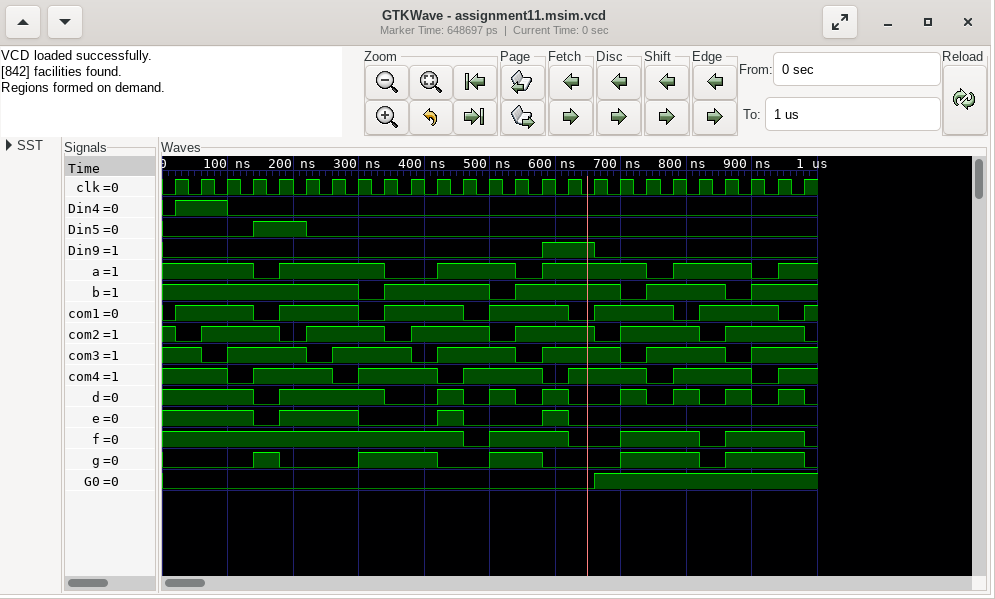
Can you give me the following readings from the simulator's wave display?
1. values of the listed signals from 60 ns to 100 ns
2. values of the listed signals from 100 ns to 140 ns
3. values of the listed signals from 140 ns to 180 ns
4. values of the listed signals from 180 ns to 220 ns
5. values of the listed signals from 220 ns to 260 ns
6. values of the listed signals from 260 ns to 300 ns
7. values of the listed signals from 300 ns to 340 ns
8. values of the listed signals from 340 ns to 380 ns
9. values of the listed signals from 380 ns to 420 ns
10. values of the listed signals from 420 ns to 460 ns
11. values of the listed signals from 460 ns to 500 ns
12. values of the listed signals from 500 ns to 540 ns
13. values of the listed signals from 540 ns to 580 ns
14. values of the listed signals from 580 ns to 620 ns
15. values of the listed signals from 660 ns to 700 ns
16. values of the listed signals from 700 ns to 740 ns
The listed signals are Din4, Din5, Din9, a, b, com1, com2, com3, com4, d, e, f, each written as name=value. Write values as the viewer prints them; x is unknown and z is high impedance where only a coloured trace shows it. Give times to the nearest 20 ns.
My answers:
Din4=1, Din5=0, Din9=0, a=1, b=1, com1=1, com2=1, com3=0, com4=1, d=1, e=1, f=1
Din4=0, Din5=0, Din9=0, a=1, b=1, com1=1, com2=1, com3=1, com4=0, d=1, e=1, f=1
Din4=0, Din5=1, Din9=0, a=0, b=1, com1=0, com2=1, com3=1, com4=1, d=0, e=0, f=1
Din4=0, Din5=1, Din9=0, a=1, b=1, com1=1, com2=0, com3=1, com4=1, d=1, e=1, f=1
Din4=0, Din5=0, Din9=0, a=1, b=1, com1=1, com2=1, com3=0, com4=1, d=1, e=1, f=1
Din4=0, Din5=0, Din9=0, a=1, b=1, com1=1, com2=1, com3=1, com4=0, d=1, e=1, f=1
Din4=0, Din5=0, Din9=0, a=1, b=0, com1=0, com2=1, com3=1, com4=1, d=1, e=0, f=1
Din4=0, Din5=0, Din9=0, a=0, b=1, com1=1, com2=0, com3=1, com4=1, d=0, e=0, f=1
Din4=0, Din5=0, Din9=0, a=0, b=1, com1=1, com2=1, com3=0, com4=1, d=0, e=0, f=1
Din4=0, Din5=0, Din9=0, a=1, b=1, com1=1, com2=1, com3=1, com4=0, d=1, e=1, f=1
Din4=0, Din5=0, Din9=0, a=1, b=1, com1=0, com2=1, com3=1, com4=1, d=0, e=0, f=0
Din4=0, Din5=0, Din9=0, a=1, b=0, com1=1, com2=0, com3=1, com4=1, d=1, e=0, f=1
Din4=0, Din5=0, Din9=0, a=0, b=1, com1=1, com2=1, com3=0, com4=1, d=0, e=0, f=1
Din4=0, Din5=0, Din9=1, a=1, b=1, com1=1, com2=1, com3=1, com4=0, d=1, e=1, f=1
Din4=0, Din5=0, Din9=0, a=1, b=1, com1=1, com2=0, com3=1, com4=1, d=0, e=0, f=0
Din4=0, Din5=0, Din9=0, a=1, b=0, com1=1, com2=1, com3=0, com4=1, d=1, e=0, f=1
